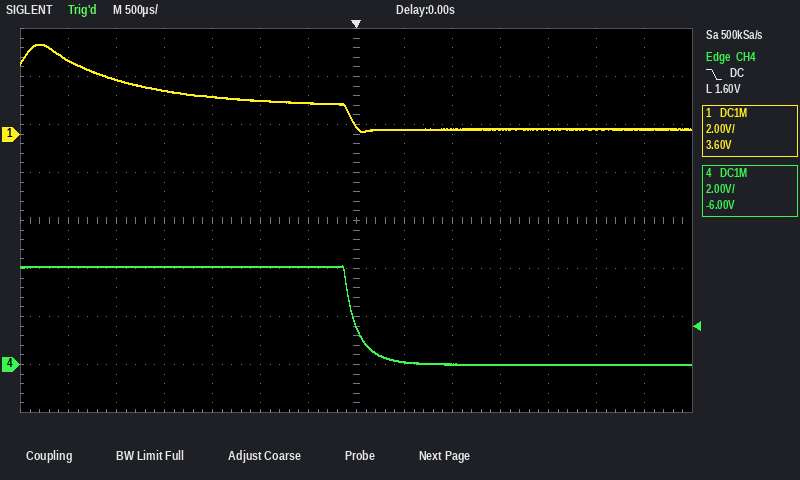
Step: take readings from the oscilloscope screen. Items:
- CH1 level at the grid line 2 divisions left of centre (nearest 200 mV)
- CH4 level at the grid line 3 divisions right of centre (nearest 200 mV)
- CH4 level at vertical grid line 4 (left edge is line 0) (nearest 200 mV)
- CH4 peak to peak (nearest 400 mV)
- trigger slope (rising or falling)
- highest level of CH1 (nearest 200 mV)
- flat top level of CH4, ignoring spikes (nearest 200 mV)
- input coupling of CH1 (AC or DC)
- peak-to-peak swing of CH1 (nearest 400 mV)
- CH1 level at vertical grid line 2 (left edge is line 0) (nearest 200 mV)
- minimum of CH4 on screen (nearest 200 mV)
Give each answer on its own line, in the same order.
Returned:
1.4 V
0.0 V
4.0 V
4.0 V
falling
3.8 V
4.0 V
DC
3.6 V
2.2 V
0.0 V
